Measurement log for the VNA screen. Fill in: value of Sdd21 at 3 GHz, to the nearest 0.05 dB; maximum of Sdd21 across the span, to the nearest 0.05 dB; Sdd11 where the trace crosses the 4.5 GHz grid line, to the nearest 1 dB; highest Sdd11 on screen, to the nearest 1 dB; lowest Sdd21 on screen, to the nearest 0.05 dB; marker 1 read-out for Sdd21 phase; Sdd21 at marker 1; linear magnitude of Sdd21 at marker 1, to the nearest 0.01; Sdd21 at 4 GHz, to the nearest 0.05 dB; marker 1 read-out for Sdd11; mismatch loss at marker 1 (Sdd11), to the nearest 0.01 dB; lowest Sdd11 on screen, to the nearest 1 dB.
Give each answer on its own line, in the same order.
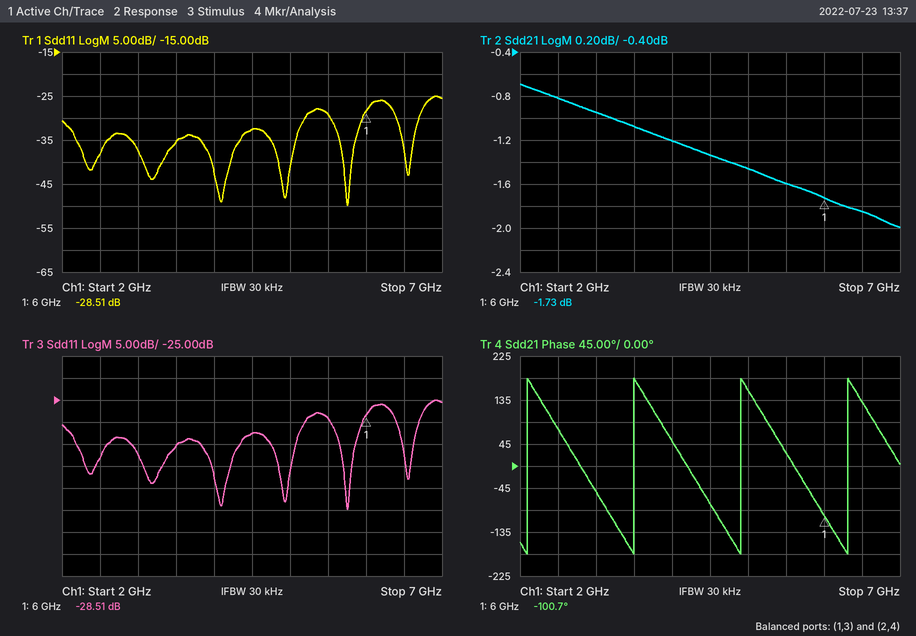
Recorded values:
-0.95 dB
-0.70 dB
-33 dB
-25 dB
-2.00 dB
-100.7°
-1.73 dB
0.82
-1.20 dB
-28.51 dB
0.01 dB
-50 dB
